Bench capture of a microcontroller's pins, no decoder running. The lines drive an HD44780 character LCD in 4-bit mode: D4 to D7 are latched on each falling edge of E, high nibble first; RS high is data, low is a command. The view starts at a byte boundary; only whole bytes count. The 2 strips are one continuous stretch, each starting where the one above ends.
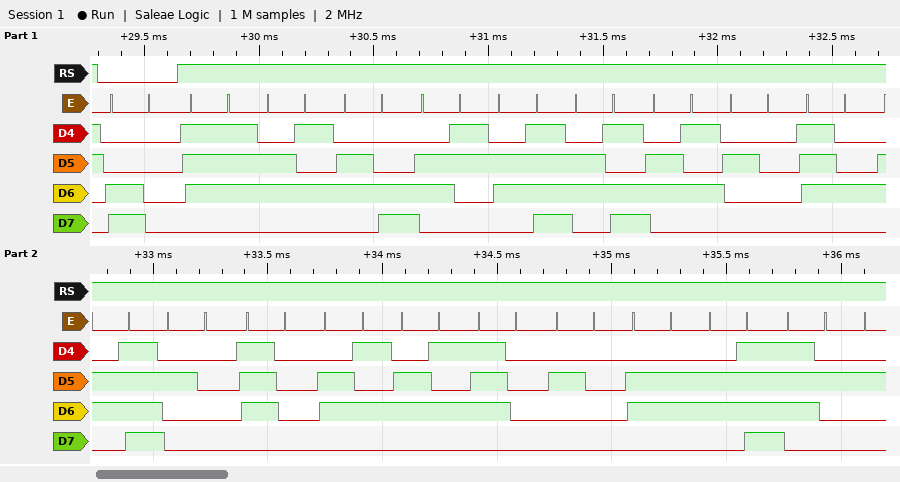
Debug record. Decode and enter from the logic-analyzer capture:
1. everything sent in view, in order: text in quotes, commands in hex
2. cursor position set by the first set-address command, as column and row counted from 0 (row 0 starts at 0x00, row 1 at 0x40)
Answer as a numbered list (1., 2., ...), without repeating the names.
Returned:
1. 0xC0 "welcome to peep for"
2. column 0, row 1
